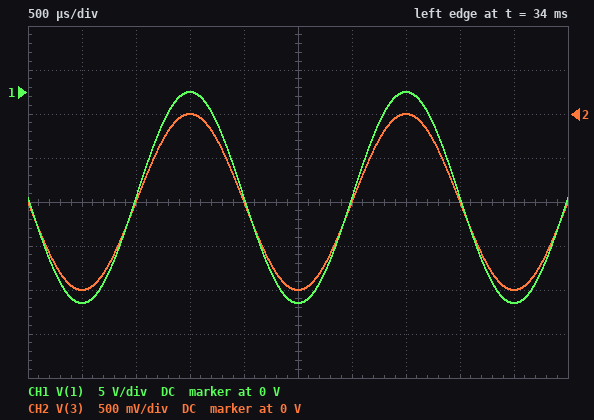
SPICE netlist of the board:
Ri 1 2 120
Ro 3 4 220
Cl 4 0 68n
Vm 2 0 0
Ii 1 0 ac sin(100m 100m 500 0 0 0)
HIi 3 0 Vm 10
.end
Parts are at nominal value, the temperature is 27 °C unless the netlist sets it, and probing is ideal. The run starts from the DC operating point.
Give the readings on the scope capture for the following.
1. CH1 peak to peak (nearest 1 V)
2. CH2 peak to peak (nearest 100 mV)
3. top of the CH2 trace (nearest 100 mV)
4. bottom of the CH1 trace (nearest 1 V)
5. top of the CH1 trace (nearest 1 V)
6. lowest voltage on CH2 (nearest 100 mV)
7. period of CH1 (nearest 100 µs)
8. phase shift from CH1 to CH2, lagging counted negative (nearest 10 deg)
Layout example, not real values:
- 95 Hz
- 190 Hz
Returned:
- 24 V
- 2.0 V
- 0 V
- -24 V
- 0 V
- -2.0 V
- 2.0 ms
- 0 deg
